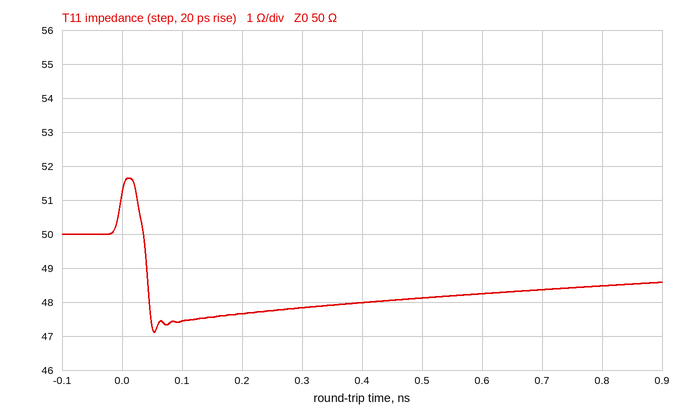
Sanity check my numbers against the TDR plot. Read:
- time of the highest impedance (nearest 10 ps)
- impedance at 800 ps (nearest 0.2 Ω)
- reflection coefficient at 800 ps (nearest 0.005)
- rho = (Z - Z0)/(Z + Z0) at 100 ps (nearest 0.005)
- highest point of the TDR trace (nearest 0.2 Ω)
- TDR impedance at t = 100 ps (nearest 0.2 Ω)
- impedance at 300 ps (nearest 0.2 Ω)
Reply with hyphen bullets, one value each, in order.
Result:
- 10 ps
- 48.4 Ω
- -0.015
- -0.025
- 51.6 Ω
- 47.4 Ω
- 47.8 Ω
